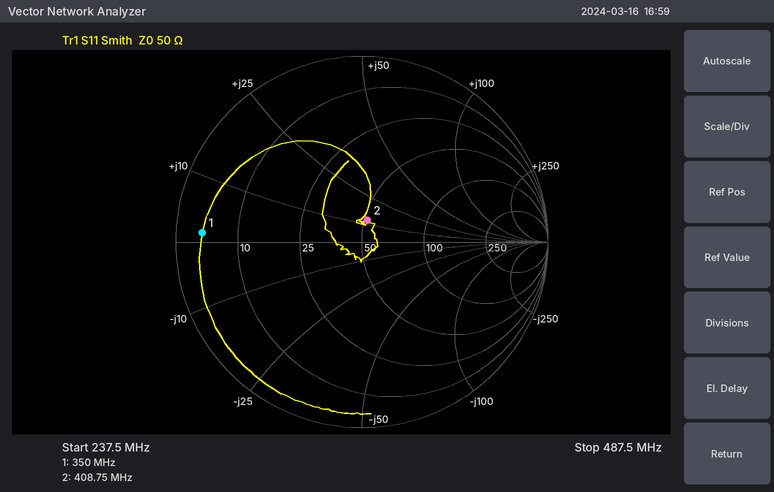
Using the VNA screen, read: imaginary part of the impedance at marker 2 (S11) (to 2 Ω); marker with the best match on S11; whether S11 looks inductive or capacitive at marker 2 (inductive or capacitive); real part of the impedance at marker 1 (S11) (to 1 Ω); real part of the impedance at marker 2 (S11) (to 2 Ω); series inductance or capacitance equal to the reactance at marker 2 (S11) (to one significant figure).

+12 Ω
marker 2
inductive
4 Ω
52 Ω
5 nH
